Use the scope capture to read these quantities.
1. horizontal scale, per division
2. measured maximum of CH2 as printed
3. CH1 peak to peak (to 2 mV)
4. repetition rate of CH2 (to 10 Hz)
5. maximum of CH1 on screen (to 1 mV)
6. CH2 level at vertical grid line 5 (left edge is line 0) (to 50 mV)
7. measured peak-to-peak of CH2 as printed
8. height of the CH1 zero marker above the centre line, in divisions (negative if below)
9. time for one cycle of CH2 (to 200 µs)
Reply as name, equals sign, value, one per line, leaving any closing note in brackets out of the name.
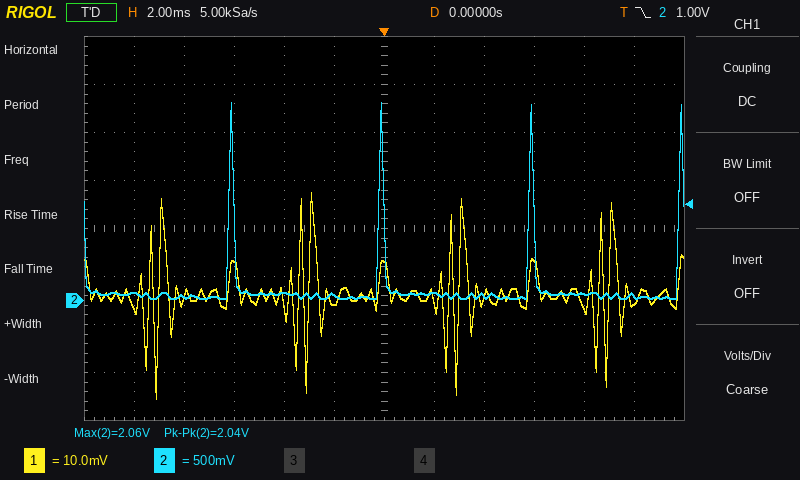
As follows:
horizontal scale, per division = 2 ms
measured maximum of CH2 as printed = 2.06 V
CH1 peak to peak = 42 mV
repetition rate of CH2 = 170 Hz
maximum of CH1 on screen = 22 mV
CH2 level at vertical grid line 5 (left edge is line 0) = 50 mV
measured peak-to-peak of CH2 as printed = 2.04 V
height of the CH1 zero marker above the centre line, in divisions = -1.5 div
time for one cycle of CH2 = 6.0 ms
